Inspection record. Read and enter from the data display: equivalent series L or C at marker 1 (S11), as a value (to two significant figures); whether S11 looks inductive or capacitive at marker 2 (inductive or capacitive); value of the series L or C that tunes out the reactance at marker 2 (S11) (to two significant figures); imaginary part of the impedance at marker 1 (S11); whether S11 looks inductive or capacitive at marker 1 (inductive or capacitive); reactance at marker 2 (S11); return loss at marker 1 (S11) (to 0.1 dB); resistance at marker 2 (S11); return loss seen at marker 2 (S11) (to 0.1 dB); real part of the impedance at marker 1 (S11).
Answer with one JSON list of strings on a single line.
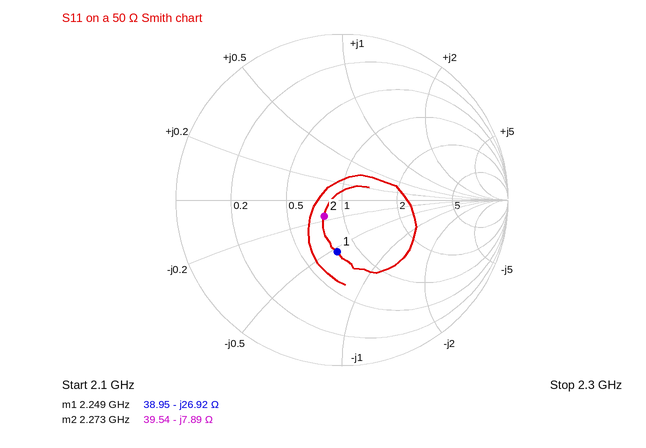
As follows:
["2.6 pF", "capacitive", "550 pH", "-26.92 Ω", "capacitive", "-7.89 Ω", "10.1 dB", "39.54 Ω", "16.7 dB", "38.95 Ω"]
